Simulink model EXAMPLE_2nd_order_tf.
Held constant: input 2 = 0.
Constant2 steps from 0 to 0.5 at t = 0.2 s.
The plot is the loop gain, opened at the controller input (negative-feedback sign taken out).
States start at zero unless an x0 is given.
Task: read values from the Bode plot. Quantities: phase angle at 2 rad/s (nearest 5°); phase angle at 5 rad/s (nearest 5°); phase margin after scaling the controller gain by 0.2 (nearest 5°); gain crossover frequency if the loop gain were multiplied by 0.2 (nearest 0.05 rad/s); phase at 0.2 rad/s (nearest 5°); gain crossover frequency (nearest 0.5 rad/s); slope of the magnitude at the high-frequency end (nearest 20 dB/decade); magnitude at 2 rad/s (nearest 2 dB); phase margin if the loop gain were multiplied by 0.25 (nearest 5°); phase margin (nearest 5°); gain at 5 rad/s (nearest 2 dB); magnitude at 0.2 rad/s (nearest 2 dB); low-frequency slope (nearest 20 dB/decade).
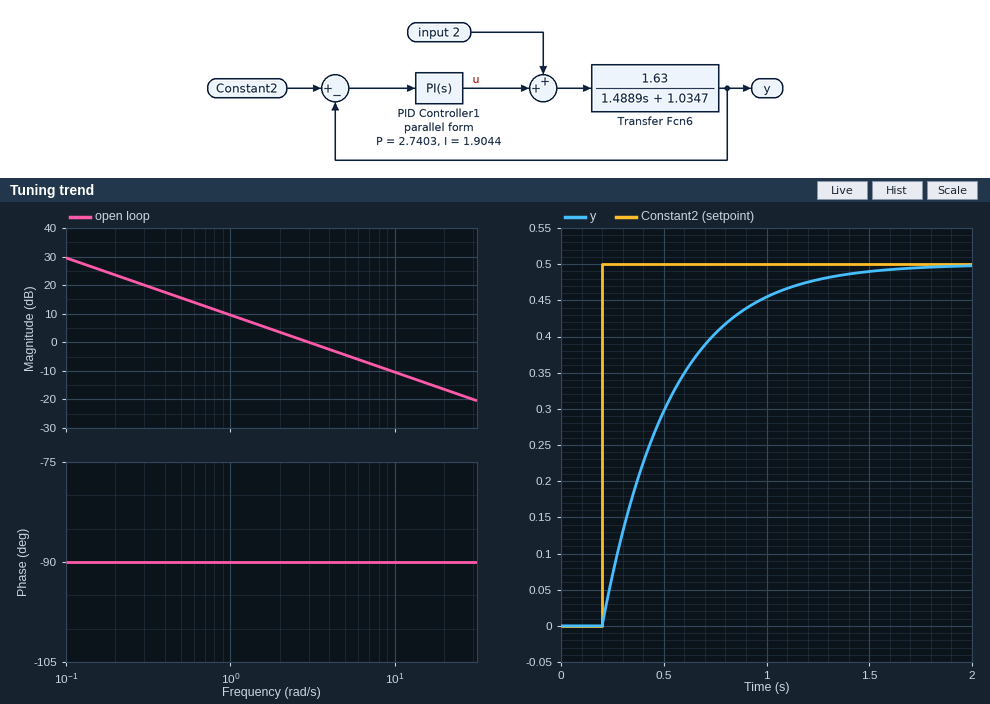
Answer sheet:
-90°
-90°
90°
0.60 rad/s
-90°
3.0 rad/s
-20 dB/decade
4 dB
90°
90°
-4 dB
24 dB
-20 dB/decade
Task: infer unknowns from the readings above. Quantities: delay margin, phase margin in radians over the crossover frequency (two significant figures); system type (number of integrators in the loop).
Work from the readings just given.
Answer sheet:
0.52 s
1
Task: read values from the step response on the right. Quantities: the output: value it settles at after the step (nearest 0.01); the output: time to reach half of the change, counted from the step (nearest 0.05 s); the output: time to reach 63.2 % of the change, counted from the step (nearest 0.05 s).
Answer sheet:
0.50
0.25 s
0.35 s
